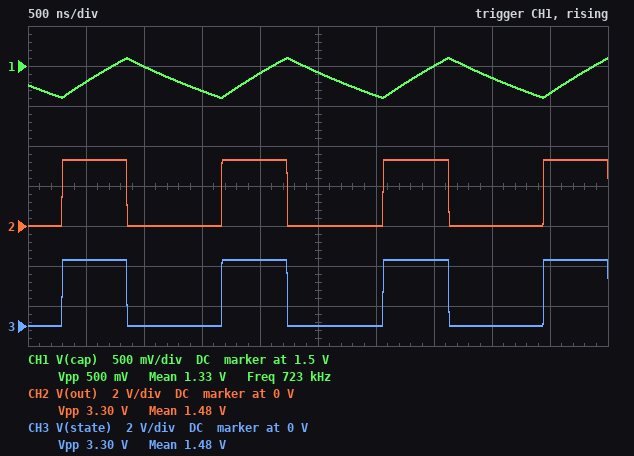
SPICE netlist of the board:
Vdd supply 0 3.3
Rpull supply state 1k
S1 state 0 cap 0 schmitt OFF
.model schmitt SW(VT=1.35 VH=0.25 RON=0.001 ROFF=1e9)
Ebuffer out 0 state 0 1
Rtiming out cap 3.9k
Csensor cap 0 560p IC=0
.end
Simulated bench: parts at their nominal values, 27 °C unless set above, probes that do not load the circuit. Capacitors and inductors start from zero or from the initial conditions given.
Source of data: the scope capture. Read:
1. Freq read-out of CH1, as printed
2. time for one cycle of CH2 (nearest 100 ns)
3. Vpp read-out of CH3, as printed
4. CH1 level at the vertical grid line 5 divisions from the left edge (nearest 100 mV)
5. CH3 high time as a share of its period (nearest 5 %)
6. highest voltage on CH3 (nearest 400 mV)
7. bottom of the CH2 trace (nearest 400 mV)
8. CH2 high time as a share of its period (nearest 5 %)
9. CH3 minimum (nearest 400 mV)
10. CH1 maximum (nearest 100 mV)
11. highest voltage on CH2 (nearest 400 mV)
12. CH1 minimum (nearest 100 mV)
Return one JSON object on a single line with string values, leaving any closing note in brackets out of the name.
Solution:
{"Freq read-out of CH1, as printed": "723 kHz", "time for one cycle of CH2": "1.4 µs", "Vpp read-out of CH3, as printed": "3.30 V", "CH1 level at the vertical grid line 5 divisions from the left edge": "1.4 V", "CH3 high time as a share of its period": "40 %", "highest voltage on CH3": "3.2 V", "bottom of the CH2 trace": "0 V", "CH2 high time as a share of its period": "40 %", "CH3 minimum": "0 V", "CH1 maximum": "1.6 V", "highest voltage on CH2": "3.2 V", "CH1 minimum": "1.1 V"}
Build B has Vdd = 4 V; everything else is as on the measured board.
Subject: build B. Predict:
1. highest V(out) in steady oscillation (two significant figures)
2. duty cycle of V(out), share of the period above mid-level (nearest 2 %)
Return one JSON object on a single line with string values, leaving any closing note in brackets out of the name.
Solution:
{"highest V(out) in steady oscillation": "4.0 V", "duty cycle of V(out), share of the period above mid-level": "34 %"}
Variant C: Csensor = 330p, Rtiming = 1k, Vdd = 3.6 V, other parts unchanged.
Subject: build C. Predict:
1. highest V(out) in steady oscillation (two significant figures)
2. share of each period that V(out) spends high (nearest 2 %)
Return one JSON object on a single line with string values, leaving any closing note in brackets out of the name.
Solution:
{"highest V(out) in steady oscillation": "3.6 V", "share of each period that V(out) spends high": "38 %"}
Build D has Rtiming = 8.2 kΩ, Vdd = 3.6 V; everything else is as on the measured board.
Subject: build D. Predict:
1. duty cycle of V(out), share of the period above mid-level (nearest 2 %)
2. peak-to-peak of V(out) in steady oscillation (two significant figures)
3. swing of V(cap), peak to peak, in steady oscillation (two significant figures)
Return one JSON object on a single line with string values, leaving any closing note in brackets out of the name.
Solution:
{"duty cycle of V(out), share of the period above mid-level": "38 %", "peak-to-peak of V(out) in steady oscillation": "3.6 V", "swing of V(cap), peak to peak, in steady oscillation": "500 mV"}
